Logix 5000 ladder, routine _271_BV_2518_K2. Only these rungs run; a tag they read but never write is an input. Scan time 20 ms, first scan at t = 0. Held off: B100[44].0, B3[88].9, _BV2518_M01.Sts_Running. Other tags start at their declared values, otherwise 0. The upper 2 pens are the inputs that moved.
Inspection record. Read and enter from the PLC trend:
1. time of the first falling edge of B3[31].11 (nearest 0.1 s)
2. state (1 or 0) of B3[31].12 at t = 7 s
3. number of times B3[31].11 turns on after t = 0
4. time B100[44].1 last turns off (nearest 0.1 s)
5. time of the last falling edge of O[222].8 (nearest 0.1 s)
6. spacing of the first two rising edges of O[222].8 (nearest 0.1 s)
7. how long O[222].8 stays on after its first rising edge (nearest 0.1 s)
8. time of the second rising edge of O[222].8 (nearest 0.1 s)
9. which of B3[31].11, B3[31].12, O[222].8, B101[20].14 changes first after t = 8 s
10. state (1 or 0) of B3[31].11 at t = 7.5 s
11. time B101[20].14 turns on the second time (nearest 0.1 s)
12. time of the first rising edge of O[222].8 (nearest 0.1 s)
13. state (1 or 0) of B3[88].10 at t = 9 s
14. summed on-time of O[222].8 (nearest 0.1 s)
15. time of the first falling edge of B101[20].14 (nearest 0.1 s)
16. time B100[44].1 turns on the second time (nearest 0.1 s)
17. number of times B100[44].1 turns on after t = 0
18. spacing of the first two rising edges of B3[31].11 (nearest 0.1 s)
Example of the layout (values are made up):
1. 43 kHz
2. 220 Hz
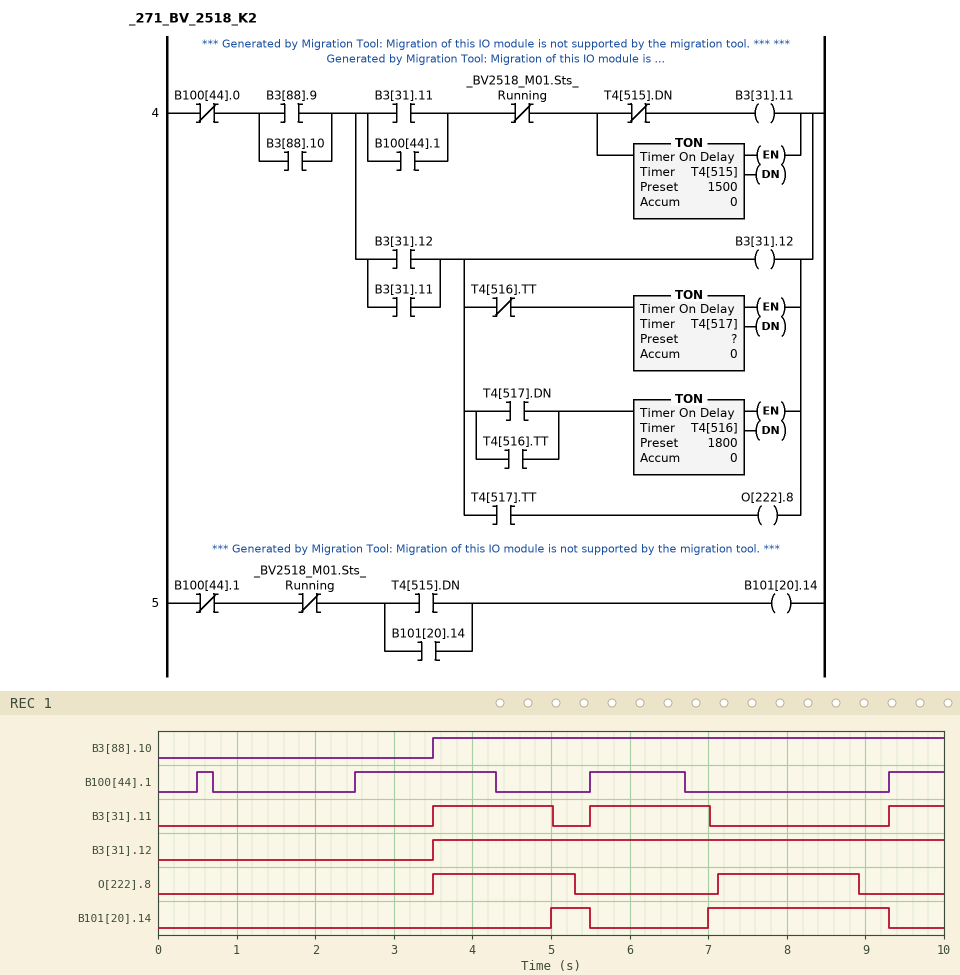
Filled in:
1. 5.0 s
2. 1
3. 3
4. 6.7 s
5. 8.9 s
6. 3.6 s
7. 1.8 s
8. 7.1 s
9. O[222].8
10. 0
11. 7.0 s
12. 3.5 s
13. 1
14. 3.6 s
15. 5.5 s
16. 2.5 s
17. 4
18. 2.0 s
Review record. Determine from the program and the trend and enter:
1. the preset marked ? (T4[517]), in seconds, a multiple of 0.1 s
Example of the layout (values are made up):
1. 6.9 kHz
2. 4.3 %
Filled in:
1. 1.8 s
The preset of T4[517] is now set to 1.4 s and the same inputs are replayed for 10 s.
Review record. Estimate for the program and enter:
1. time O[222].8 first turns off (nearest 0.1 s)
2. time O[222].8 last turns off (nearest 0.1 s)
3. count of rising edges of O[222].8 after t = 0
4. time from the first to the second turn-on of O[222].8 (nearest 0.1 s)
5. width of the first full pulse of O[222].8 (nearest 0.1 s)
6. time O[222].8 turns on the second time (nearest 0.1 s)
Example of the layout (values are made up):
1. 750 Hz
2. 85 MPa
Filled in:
1. 4.9 s
2. 8.1 s
3. 3
4. 3.2 s
5. 1.4 s
6. 6.7 s
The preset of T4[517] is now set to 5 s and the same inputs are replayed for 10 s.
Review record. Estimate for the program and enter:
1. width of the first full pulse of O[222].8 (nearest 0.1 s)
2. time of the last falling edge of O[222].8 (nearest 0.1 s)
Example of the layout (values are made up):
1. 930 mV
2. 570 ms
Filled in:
1. 5.0 s
2. 8.5 s
